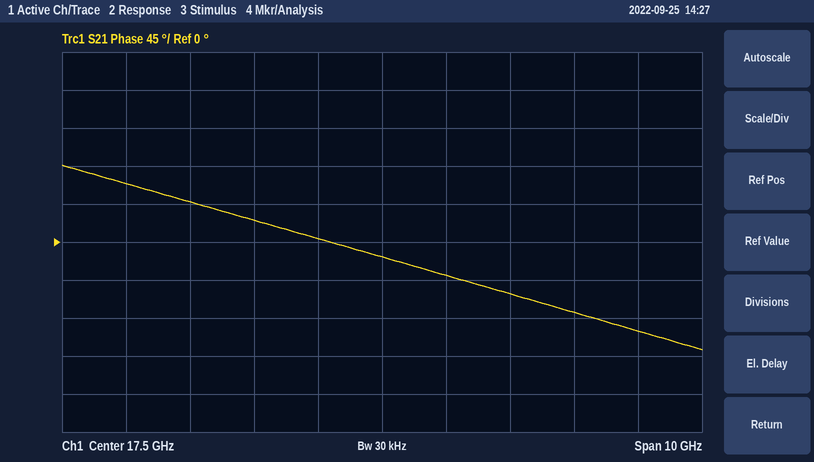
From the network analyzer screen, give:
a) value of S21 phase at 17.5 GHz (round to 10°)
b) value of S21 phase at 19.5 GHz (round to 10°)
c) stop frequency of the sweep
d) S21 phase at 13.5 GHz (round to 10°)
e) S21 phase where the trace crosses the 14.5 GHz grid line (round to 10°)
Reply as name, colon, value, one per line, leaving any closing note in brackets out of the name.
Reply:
value of S21 phase at 17.5 GHz: -20°
value of S21 phase at 19.5 GHz: -60°
stop frequency of the sweep: 22.5 GHz
S21 phase at 13.5 GHz: 70°
S21 phase where the trace crosses the 14.5 GHz grid line: 50°
